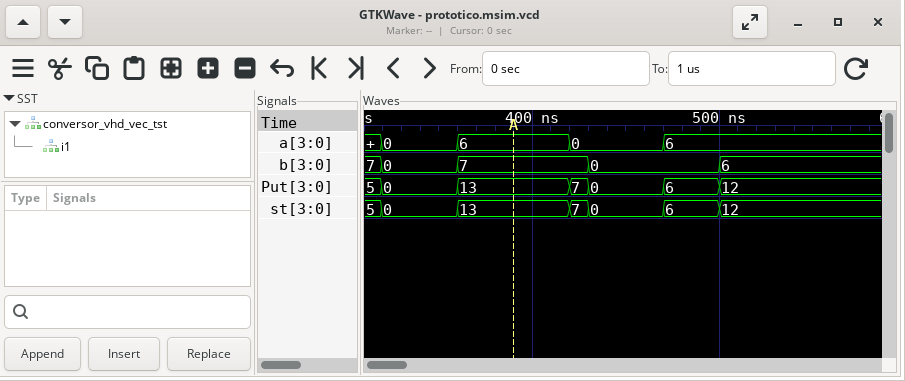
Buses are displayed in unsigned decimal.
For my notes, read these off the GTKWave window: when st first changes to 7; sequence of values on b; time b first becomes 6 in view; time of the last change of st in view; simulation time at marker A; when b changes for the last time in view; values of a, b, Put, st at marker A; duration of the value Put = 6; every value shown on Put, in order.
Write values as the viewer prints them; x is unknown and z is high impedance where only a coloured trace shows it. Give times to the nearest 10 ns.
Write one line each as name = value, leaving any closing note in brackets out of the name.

when st first changes to 7 = 420 ns
sequence of values on b = 7, 0, 7, 0, 6
time b first becomes 6 in view = 500 ns
time of the last change of st in view = 500 ns
simulation time at marker A = 390 ns
when b changes for the last time in view = 500 ns
values of a, b, Put, st at marker A = a=6, b=7, Put=13, st=13
duration of the value Put = 6 = 30 ns
every value shown on Put, in order = 5, 0, 13, 7, 0, 6, 12
